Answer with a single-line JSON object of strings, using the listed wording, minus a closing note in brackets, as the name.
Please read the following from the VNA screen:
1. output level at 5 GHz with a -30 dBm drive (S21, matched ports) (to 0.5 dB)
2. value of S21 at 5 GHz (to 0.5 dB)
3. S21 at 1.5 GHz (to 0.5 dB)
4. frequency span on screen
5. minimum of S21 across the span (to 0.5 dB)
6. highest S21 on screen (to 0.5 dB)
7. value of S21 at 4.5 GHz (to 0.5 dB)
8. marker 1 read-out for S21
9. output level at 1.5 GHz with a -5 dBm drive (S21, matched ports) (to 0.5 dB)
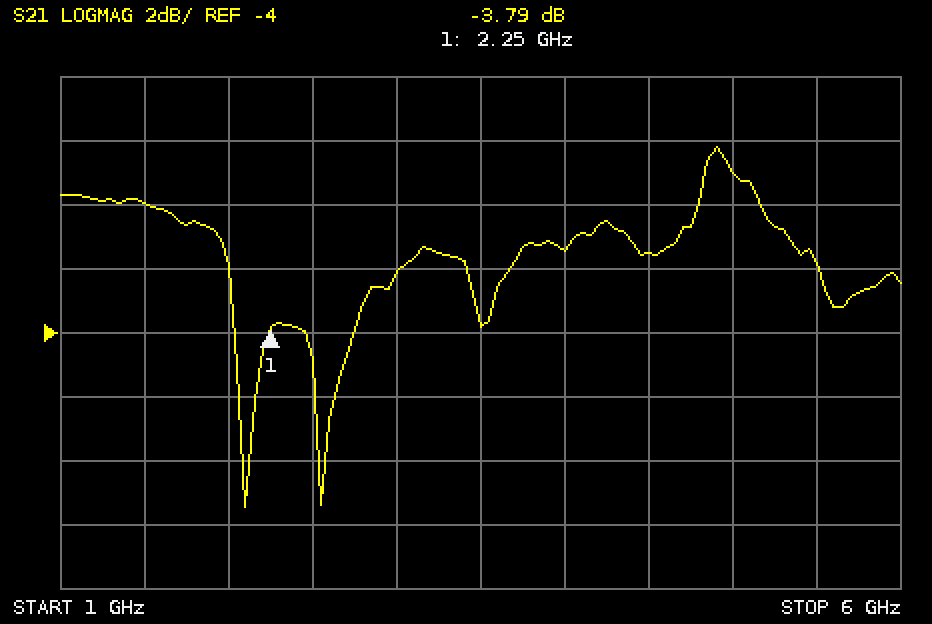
{"output level at 5 GHz with a -30 dBm drive (S21, matched ports)": "-29.0 dBm", "value of S21 at 5 GHz": "1.0 dB", "S21 at 1.5 GHz": "0.0 dB", "frequency span on screen": "5 GHz", "minimum of S21 across the span": "-9.5 dB", "highest S21 on screen": "2.0 dB", "value of S21 at 4.5 GHz": "-1.5 dB", "marker 1 read-out for S21": "-3.79 dB", "output level at 1.5 GHz with a -5 dBm drive (S21, matched ports)": "-5.0 dBm"}
